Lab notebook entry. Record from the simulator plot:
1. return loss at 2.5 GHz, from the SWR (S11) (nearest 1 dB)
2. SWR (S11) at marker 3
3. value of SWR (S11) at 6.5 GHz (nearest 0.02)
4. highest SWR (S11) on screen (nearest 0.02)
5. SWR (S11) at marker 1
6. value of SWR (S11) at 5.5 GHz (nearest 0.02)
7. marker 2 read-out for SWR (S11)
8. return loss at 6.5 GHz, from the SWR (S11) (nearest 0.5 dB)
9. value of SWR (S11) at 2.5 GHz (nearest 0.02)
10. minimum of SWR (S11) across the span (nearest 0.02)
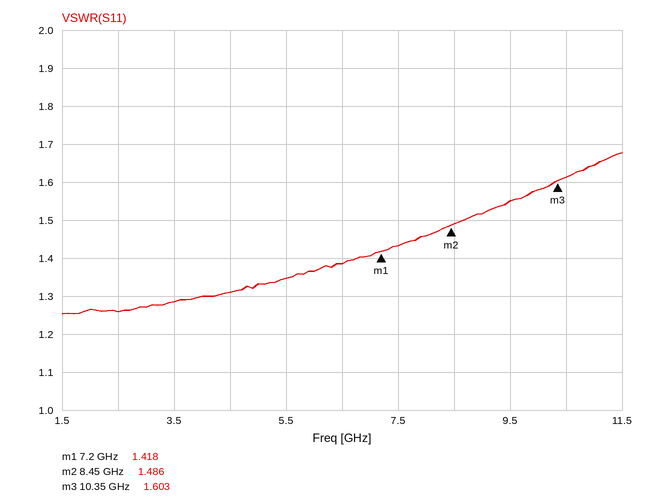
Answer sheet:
19 dB
1.603
1.38
1.68
1.418
1.34
1.486
16.0 dB
1.26
1.26
